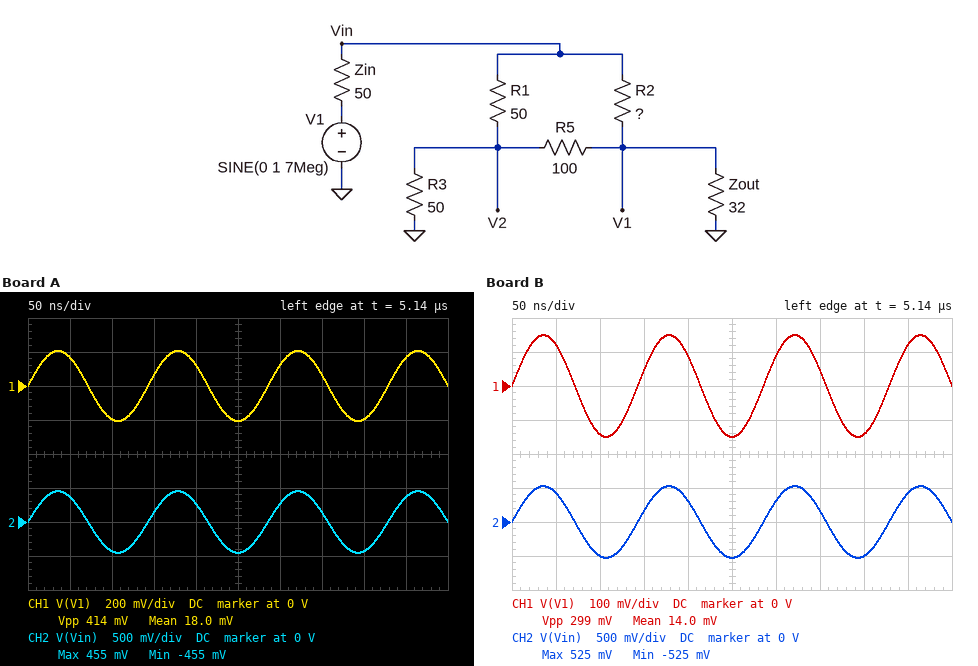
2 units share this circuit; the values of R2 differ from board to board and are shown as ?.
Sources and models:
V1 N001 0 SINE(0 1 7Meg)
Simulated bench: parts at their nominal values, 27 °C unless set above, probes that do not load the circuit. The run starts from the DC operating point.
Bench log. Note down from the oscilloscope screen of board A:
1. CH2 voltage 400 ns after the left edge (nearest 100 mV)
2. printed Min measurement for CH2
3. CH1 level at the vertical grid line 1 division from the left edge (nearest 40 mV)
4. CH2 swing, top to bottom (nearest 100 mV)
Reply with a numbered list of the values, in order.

1. -400 mV
2. -455 mV
3. 160 mV
4. 900 mV
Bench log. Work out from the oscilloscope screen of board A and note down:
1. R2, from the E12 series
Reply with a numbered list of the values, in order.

1. 39 Ω
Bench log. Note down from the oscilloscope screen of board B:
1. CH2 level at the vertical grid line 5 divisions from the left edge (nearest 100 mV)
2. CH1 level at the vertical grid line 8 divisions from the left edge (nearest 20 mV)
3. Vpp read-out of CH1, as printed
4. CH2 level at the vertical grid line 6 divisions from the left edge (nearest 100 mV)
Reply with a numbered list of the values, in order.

1. -500 mV
2. -140 mV
3. 299 mV
4. 300 mV
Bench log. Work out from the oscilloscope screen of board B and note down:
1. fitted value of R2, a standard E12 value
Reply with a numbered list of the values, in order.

1. 100 Ω
